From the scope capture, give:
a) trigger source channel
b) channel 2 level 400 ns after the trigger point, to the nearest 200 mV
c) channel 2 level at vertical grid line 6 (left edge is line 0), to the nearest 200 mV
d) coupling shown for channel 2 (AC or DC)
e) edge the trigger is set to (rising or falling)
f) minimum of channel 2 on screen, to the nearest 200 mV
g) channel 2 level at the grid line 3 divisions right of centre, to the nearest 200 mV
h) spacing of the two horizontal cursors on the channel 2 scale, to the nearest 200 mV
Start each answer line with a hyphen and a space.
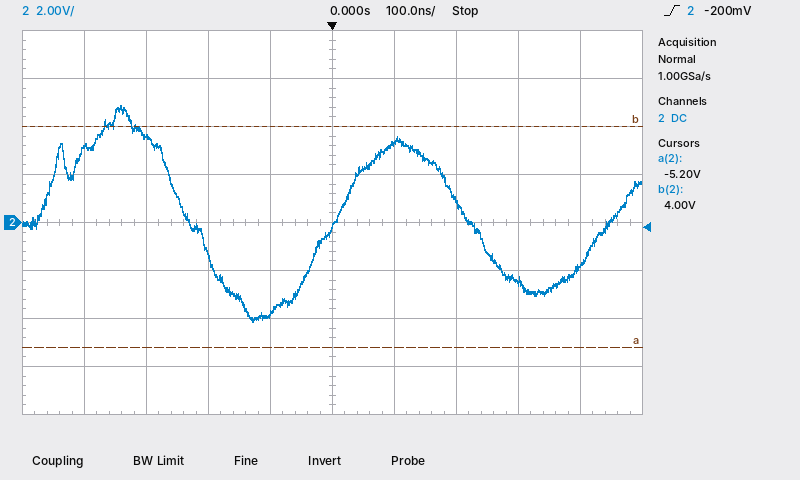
- channel 2
- -1.8 V
- 3.4 V
- DC
- rising
- -4.2 V
- -2.4 V
- 9.2 V
